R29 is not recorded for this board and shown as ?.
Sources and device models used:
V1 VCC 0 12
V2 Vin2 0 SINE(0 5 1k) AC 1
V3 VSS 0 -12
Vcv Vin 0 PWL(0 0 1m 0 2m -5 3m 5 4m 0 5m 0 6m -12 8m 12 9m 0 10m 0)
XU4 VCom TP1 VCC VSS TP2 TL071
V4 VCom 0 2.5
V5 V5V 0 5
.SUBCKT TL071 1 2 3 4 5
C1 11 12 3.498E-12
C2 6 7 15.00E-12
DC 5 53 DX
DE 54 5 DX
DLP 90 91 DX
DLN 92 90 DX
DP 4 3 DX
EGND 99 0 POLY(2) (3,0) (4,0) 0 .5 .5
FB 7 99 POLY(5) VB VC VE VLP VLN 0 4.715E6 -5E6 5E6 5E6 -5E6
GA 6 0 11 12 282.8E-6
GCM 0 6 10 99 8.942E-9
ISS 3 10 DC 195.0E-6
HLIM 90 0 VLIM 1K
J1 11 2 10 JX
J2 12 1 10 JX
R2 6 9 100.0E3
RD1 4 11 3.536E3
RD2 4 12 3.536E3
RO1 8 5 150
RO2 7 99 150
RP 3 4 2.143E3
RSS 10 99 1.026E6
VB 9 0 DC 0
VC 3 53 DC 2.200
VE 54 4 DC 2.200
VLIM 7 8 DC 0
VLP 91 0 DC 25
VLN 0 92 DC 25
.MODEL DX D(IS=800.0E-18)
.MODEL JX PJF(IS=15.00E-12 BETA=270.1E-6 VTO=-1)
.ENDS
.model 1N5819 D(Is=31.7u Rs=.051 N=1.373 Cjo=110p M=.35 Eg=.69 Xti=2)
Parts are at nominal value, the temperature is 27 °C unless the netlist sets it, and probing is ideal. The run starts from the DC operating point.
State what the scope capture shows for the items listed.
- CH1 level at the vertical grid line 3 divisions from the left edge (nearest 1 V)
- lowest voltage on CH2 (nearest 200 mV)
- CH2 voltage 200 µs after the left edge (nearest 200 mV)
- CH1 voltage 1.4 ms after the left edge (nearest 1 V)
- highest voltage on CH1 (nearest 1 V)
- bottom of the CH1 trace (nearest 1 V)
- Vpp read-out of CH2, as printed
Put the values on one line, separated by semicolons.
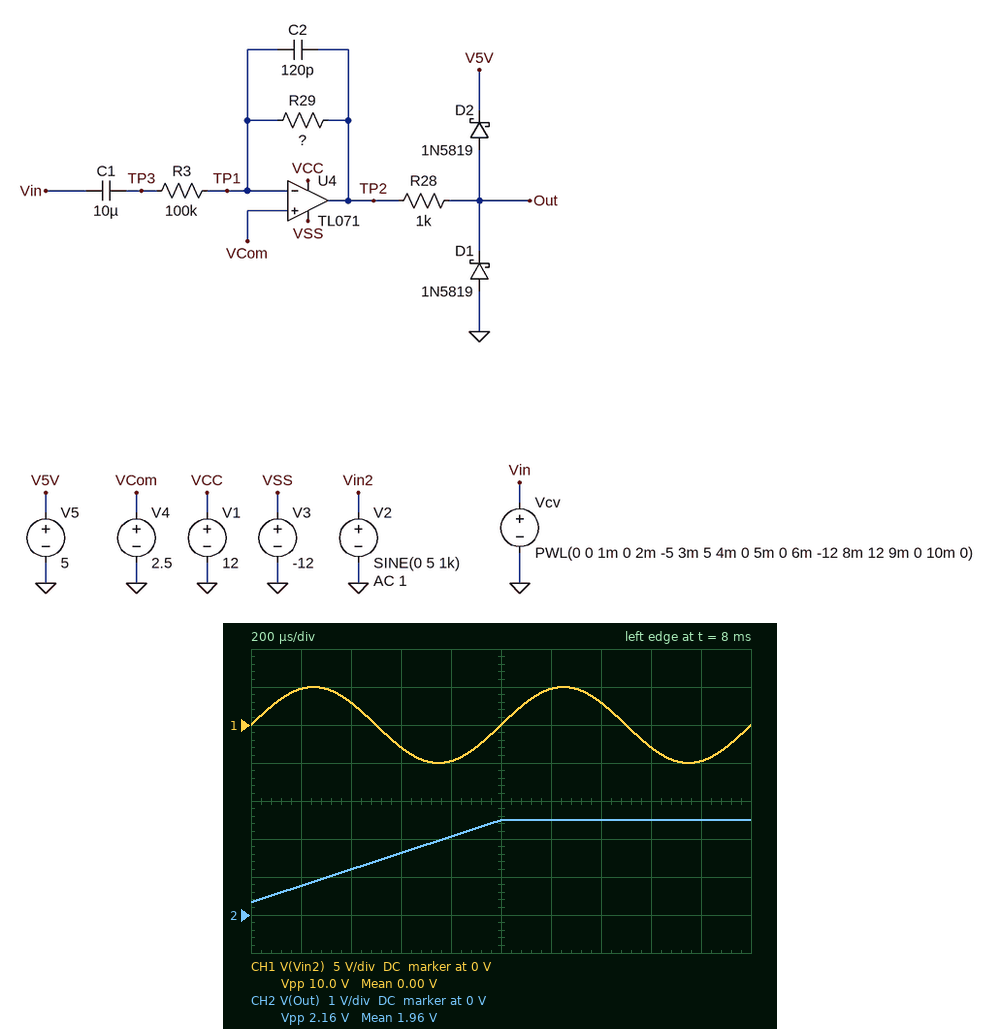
-3 V; 400 mV; 800 mV; 3 V; 5 V; -5 V; 2.16 V
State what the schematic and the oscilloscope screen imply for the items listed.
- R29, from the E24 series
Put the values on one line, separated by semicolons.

18 kΩ
